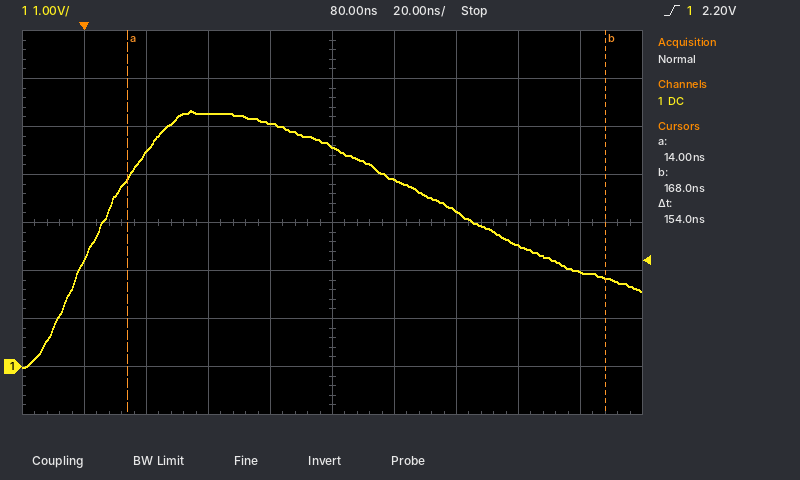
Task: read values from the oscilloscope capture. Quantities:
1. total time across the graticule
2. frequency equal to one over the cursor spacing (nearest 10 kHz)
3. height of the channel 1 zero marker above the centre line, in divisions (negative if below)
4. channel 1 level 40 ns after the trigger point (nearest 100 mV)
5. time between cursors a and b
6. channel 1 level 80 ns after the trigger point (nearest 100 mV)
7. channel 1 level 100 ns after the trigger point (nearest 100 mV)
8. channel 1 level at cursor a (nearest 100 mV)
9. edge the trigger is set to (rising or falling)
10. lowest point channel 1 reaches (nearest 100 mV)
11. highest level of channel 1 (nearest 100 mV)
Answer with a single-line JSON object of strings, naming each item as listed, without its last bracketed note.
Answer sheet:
{"total time across the graticule": "200 ns", "frequency equal to one over the cursor spacing": "6.49 MHz", "height of the channel 1 zero marker above the centre line, in divisions": "-3.0 div", "channel 1 level 40 ns after the trigger point": "5.3 V", "time between cursors a and b": "154 ns", "channel 1 level 80 ns after the trigger point": "4.6 V", "channel 1 level 100 ns after the trigger point": "3.9 V", "channel 1 level at cursor a": "3.9 V", "edge the trigger is set to": "rising", "lowest point channel 1 reaches": "0.0 V", "highest level of channel 1": "5.3 V"}
